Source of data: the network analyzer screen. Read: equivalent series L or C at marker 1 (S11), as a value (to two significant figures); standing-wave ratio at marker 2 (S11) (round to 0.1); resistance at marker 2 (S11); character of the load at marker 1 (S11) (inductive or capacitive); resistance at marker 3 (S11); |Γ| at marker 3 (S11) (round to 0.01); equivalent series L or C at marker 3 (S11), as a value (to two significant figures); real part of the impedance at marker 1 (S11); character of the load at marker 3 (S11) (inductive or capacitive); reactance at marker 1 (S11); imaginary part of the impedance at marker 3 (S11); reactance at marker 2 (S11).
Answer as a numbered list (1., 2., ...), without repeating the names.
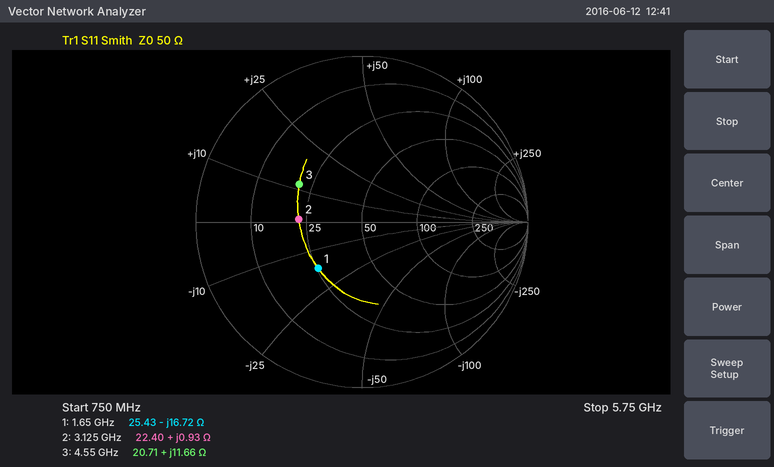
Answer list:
1. 5.8 pF
2. 2.2
3. 22.40 Ω
4. capacitive
5. 20.71 Ω
6. 0.44
7. 410 pH
8. 25.43 Ω
9. inductive
10. -16.72 Ω
11. +11.66 Ω
12. +0.93 Ω
